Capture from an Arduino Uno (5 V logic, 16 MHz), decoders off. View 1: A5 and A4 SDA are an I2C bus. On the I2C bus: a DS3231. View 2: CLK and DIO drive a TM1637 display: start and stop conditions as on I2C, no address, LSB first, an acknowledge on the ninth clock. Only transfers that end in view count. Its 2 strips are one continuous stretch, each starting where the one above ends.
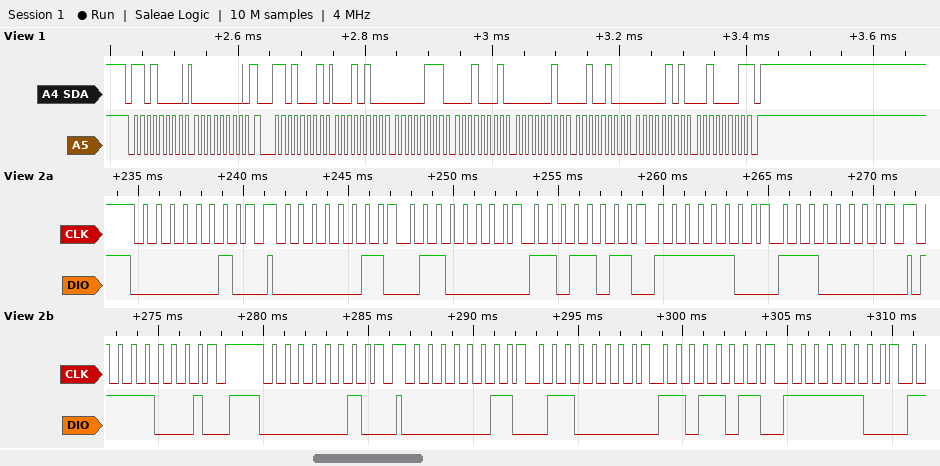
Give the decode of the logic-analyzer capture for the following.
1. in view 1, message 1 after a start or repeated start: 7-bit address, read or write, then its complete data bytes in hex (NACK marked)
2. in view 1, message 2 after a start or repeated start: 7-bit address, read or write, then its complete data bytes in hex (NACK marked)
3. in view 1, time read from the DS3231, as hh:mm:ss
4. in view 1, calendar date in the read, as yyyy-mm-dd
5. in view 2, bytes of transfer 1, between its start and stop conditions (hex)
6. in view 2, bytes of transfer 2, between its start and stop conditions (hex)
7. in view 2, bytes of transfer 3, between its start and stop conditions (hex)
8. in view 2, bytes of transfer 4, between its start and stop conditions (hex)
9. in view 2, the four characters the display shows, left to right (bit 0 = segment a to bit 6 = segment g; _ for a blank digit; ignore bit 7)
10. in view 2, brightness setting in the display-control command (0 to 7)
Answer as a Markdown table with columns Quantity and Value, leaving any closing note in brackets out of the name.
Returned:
| Quantity | Value |
|---|---|
| in view 1, message 1 after a start or repeated start: 7-bit address, read or write, then its complete data bytes in hex | 0x68 write: 00 |
| in view 1, message 2 after a start or repeated start: 7-bit address, read or write, then its complete data bytes in hex | 0x68 read: 14 07 11 02 24 05 21 NACK |
| in view 1, time read from the DS3231, as hh:mm:ss | 11:07:14 |
| in view 1, calendar date in the read, as yyyy-mm-dd | 2021-05-24 |
| in view 2, bytes of transfer 1, between its start and stop conditions | 40 |
| in view 2, bytes of transfer 2, between its start and stop conditions | C0 06 DB 3F 07 |
| in view 2, bytes of transfer 3, between its start and stop conditions | 8F |
| in view 2, bytes of transfer 4, between its start and stop conditions | 40 |
| in view 2, the four characters the display shows, left to right | 1207 |
| in view 2, brightness setting in the display-control command | 7 |
